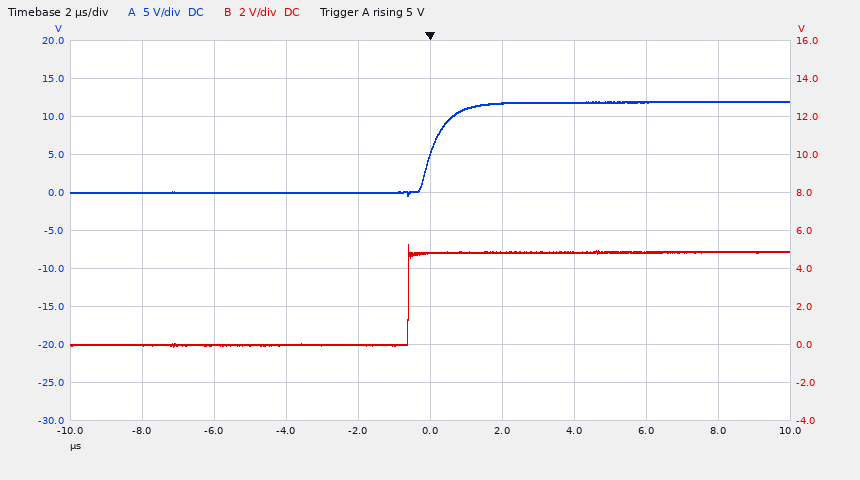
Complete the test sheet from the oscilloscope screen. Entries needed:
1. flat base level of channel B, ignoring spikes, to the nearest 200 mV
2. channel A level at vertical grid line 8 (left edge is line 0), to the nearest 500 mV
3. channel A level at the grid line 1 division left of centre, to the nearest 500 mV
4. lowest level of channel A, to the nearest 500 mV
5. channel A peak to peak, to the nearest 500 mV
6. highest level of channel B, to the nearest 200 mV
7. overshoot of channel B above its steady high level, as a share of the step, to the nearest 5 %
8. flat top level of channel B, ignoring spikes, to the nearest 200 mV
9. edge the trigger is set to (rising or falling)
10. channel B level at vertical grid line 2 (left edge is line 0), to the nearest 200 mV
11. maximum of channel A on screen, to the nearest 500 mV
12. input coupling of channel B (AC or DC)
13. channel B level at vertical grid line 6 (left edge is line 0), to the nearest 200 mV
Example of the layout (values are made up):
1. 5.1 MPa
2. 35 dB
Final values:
1. 0.0 V
2. 12.0 V
3. 0.0 V
4. -500 mV
5. 12.5 V
6. 5.2 V
7. 10 %
8. 4.8 V
9. rising
10. 0.0 V
11. 12.0 V
12. DC
13. 4.8 V
